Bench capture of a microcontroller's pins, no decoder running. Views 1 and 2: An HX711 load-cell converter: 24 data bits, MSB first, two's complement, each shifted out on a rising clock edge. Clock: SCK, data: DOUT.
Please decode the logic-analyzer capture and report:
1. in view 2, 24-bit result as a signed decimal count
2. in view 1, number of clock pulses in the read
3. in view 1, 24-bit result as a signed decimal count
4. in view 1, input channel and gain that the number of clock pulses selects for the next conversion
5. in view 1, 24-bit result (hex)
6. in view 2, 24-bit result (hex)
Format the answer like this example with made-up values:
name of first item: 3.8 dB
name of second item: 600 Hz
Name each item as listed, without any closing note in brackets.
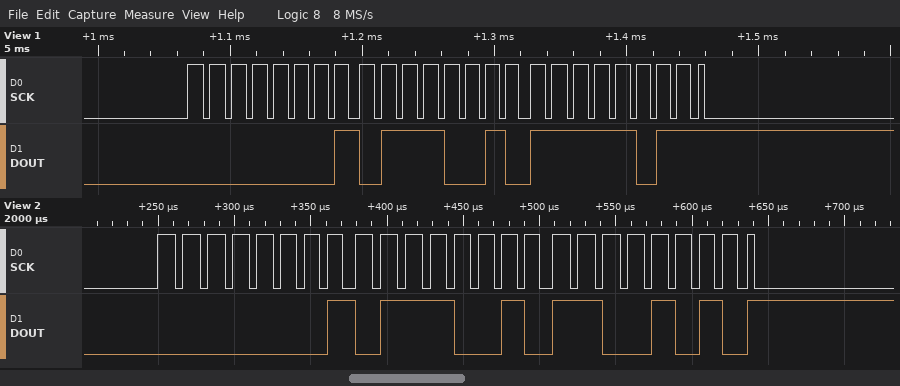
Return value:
in view 2, 24-bit result as a signed decimal count: 94922
in view 1, number of clock pulses in the read: 25
in view 1, 24-bit result as a signed decimal count: 94971
in view 1, input channel and gain that the number of clock pulses selects for the next conversion: channel A, gain 128
in view 1, 24-bit result: 0x0172FB
in view 2, 24-bit result: 0x0172CA
